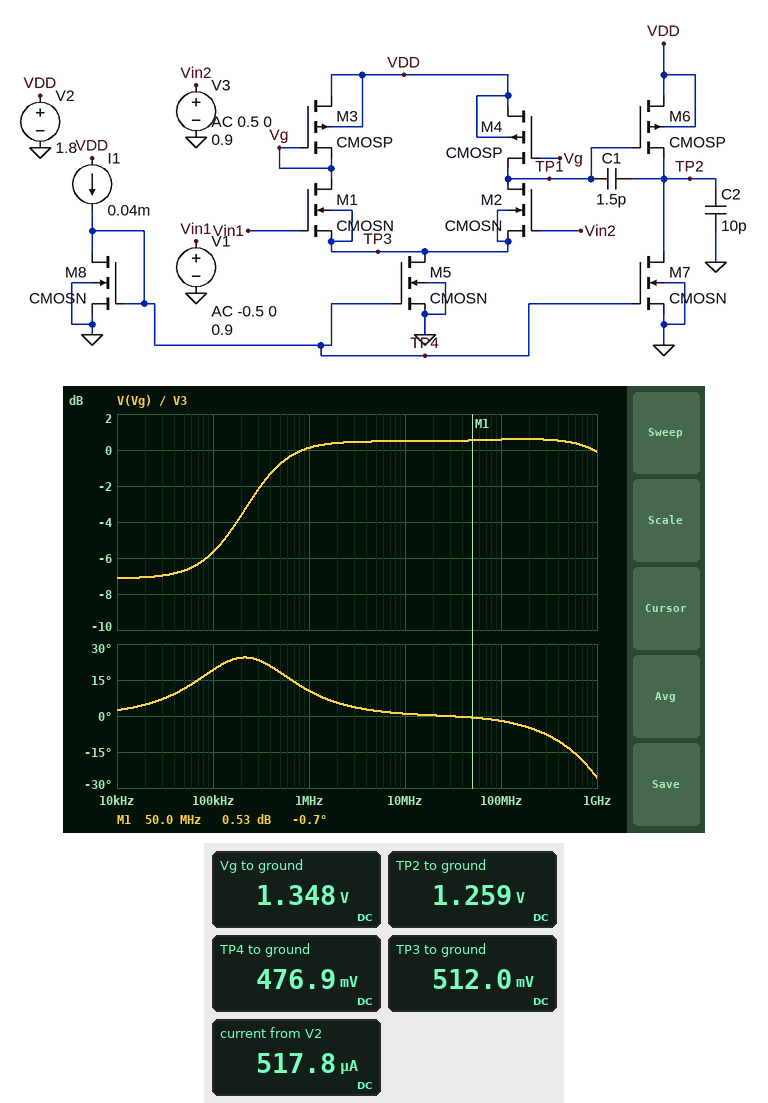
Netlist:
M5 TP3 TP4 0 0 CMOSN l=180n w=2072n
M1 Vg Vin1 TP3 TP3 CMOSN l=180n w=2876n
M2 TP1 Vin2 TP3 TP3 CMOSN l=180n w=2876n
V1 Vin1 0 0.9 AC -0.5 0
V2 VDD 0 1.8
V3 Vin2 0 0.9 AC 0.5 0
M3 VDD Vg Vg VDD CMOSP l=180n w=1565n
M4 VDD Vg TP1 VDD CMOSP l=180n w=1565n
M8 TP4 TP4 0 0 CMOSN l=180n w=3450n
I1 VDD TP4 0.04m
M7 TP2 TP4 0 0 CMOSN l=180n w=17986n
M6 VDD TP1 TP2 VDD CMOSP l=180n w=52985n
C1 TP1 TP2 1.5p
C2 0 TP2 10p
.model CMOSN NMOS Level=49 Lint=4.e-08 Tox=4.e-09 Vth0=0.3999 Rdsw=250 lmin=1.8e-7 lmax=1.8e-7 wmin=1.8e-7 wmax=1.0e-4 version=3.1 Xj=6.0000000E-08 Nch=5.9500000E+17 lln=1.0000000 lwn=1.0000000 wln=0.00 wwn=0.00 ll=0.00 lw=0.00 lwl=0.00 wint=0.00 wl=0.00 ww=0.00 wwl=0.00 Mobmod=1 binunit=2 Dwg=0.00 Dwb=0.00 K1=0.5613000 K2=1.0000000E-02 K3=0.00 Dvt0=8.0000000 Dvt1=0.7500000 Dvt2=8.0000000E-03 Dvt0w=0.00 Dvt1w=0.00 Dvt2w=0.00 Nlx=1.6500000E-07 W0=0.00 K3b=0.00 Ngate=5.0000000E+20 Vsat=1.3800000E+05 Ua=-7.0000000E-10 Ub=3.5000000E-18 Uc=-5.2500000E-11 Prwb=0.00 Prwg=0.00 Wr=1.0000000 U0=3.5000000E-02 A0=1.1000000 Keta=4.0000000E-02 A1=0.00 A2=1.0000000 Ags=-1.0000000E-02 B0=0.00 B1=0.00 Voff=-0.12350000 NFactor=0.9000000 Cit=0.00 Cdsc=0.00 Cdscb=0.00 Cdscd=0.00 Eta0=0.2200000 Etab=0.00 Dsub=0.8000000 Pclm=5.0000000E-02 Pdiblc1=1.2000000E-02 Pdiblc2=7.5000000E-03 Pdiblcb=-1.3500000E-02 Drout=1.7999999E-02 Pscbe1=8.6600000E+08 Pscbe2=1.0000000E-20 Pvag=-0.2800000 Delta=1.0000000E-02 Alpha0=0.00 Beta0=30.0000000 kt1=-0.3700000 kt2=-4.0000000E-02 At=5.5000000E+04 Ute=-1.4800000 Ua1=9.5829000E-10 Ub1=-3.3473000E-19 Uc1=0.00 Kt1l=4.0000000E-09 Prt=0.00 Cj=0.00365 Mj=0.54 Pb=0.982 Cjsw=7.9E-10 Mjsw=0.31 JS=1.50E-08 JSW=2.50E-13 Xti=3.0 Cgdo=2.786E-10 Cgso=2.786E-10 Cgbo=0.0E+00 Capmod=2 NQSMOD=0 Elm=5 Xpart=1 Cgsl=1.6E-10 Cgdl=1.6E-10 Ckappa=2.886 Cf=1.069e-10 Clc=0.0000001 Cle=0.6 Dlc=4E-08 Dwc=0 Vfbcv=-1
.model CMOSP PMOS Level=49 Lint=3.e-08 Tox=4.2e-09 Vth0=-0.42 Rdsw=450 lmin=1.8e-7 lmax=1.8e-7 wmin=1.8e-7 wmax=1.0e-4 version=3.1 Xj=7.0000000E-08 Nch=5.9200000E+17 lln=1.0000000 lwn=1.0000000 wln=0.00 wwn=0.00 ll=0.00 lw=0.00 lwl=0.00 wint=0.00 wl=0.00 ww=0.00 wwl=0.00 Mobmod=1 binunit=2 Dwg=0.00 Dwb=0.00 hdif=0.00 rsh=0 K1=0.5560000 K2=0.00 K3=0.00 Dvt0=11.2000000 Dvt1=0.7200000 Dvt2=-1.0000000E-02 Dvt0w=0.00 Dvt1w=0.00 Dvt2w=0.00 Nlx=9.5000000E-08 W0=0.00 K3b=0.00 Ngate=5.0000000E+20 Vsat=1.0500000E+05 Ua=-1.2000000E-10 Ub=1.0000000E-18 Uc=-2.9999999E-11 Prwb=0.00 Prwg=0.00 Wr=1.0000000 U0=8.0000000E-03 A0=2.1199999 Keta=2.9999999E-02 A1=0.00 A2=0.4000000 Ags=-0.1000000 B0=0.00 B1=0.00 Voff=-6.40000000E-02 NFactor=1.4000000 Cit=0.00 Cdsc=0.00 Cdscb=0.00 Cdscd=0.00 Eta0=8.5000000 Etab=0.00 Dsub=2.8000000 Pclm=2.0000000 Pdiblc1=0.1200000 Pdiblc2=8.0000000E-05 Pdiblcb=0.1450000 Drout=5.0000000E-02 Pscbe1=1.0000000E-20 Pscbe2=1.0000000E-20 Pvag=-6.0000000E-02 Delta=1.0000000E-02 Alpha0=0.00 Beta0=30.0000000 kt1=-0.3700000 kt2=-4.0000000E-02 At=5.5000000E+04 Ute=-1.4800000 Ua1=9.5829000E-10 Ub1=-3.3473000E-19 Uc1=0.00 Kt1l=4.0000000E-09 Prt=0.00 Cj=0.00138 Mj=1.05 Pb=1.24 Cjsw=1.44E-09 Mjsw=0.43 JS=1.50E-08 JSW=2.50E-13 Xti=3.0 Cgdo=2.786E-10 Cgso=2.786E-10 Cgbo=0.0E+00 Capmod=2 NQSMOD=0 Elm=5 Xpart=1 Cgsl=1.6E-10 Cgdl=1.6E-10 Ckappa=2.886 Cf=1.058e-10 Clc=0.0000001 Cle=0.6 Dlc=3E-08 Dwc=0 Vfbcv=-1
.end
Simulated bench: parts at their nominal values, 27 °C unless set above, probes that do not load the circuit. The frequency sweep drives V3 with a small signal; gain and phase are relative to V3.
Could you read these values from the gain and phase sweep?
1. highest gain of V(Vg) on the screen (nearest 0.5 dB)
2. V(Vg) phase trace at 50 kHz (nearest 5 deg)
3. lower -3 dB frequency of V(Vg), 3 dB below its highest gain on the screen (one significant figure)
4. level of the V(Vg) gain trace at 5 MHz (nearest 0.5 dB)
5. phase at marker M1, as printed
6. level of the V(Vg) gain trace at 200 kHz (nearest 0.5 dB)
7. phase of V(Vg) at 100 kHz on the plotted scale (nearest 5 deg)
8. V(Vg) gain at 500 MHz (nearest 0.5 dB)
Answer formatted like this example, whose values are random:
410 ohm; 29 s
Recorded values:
0.5 dB; 10 deg; 300 kHz; 0.5 dB; -0.7 deg; -3.5 dB; 20 deg; 0.5 dB
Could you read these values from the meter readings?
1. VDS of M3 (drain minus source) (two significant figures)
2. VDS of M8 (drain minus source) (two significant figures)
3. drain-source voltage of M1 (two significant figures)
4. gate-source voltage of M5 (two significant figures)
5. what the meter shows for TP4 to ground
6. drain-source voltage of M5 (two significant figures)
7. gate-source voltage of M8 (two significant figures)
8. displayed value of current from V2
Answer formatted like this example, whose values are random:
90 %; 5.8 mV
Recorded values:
450 mV; 480 mV; 840 mV; 480 mV; 476.9 mV; 510 mV; 480 mV; 517.8 µA
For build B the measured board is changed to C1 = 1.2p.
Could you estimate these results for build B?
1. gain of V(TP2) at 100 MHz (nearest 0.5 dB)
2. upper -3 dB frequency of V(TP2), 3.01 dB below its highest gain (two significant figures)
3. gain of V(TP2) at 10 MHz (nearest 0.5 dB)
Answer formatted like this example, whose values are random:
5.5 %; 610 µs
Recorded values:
-13.0 dB; 410 kHz; 10.5 dB
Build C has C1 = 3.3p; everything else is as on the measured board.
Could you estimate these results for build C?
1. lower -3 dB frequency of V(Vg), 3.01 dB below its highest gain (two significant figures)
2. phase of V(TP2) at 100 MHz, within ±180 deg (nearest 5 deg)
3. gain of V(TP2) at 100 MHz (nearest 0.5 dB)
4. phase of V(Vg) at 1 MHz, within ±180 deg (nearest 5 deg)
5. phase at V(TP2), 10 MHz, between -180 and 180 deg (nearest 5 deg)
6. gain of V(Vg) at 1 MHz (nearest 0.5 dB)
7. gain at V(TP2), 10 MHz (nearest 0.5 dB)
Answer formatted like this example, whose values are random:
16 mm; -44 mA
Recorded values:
130 kHz; -165 deg; -21.0 dB; 5 deg; -100 deg; 0.5 dB; 2.0 dB
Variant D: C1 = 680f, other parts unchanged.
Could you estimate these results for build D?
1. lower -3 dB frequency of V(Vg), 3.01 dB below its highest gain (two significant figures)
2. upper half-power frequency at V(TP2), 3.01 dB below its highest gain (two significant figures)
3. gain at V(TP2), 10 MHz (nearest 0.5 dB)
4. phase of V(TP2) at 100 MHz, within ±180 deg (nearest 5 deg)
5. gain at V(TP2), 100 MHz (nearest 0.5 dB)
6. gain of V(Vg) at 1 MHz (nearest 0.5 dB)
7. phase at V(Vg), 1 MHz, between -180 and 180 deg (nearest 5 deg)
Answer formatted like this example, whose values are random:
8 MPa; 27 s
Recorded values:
600 kHz; 690 kHz; 15.0 dB; -145 deg; -8.5 dB; -1.0 dB; 20 deg
